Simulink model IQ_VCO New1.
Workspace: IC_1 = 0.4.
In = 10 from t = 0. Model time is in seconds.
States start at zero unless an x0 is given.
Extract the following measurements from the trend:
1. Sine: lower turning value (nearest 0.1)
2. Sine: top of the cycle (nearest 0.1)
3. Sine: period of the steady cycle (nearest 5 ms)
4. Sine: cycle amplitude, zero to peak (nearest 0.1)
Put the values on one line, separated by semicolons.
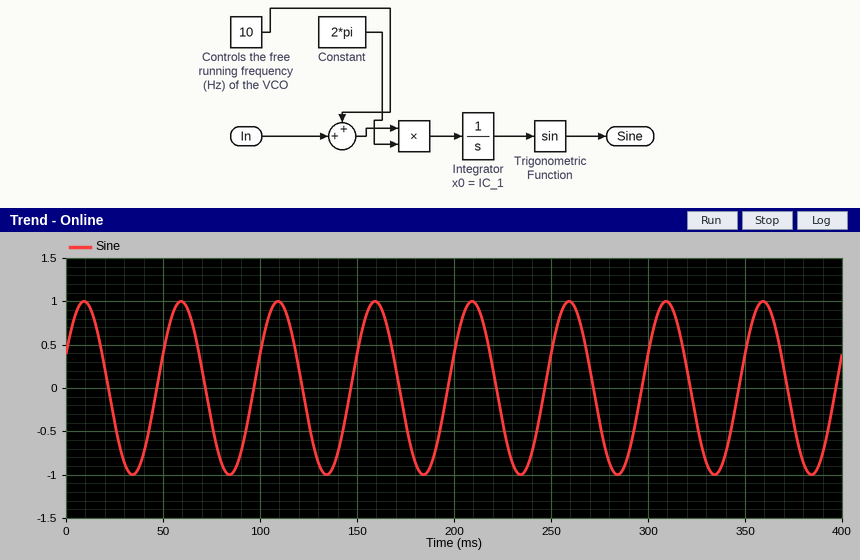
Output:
-1.0; 1.0; 50 ms; 1.0
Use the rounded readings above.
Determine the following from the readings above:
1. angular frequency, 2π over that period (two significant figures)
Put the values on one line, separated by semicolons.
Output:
0.13 rad/ms
